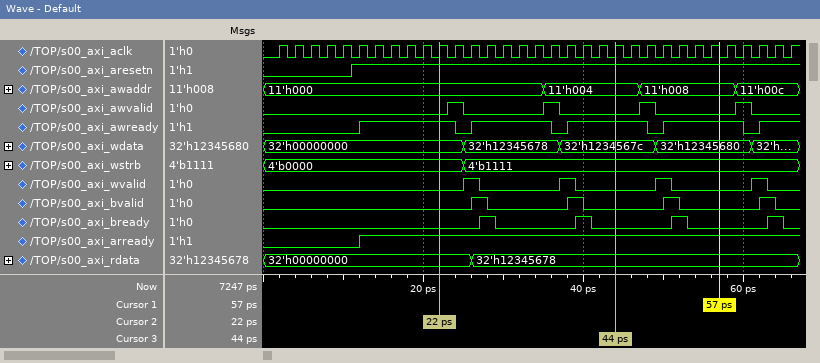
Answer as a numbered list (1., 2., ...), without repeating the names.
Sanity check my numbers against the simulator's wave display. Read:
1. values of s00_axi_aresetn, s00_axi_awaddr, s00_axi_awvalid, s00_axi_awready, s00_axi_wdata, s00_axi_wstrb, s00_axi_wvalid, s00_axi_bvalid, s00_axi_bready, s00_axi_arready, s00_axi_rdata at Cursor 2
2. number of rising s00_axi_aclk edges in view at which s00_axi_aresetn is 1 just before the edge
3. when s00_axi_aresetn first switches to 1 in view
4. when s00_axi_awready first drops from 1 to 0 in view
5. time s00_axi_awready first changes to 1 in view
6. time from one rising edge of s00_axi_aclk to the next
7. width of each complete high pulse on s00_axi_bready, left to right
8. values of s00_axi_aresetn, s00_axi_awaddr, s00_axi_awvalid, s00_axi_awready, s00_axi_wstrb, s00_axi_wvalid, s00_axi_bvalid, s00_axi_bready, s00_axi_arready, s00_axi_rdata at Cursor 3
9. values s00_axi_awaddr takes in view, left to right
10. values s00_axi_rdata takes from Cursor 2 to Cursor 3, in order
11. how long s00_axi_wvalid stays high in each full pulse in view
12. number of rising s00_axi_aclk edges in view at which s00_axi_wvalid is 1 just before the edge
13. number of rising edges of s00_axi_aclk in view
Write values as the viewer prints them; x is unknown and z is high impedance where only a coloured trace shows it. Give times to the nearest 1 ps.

1. s00_axi_aresetn=1, s00_axi_awaddr=11'h000, s00_axi_awvalid=0, s00_axi_awready=1, s00_axi_wdata=32'h00000000, s00_axi_wstrb=4'b0000, s00_axi_wvalid=0, s00_axi_bvalid=0, s00_axi_bready=0, s00_axi_arready=1, s00_axi_rdata=32'h00000000
2. 28
3. 11 ps
4. 24 ps
5. 12 ps
6. 2 ps
7. 2 ps, 2 ps, 2 ps, 2 ps
8. s00_axi_aresetn=1, s00_axi_awaddr=11'h004, s00_axi_awvalid=0, s00_axi_awready=1, s00_axi_wstrb=4'b1111, s00_axi_wvalid=0, s00_axi_bvalid=0, s00_axi_bready=0, s00_axi_arready=1, s00_axi_rdata=32'h12345678
9. 11'h000, 11'h004, 11'h008, 11'h00c
10. 32'h00000000, 32'h12345678
11. 2 ps, 2 ps, 2 ps, 2 ps
12. 4
13. 33
